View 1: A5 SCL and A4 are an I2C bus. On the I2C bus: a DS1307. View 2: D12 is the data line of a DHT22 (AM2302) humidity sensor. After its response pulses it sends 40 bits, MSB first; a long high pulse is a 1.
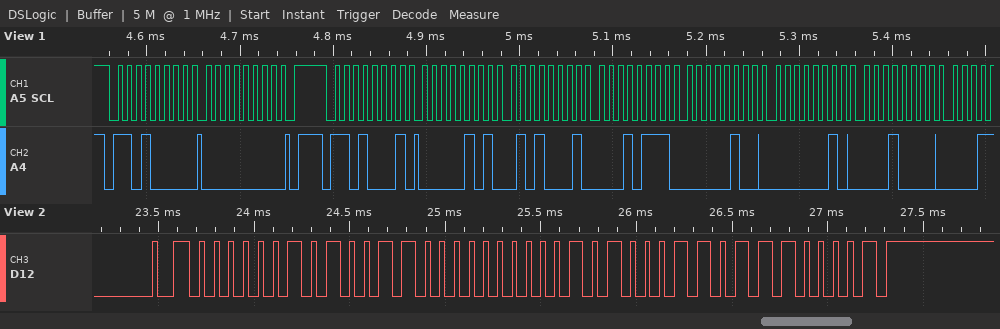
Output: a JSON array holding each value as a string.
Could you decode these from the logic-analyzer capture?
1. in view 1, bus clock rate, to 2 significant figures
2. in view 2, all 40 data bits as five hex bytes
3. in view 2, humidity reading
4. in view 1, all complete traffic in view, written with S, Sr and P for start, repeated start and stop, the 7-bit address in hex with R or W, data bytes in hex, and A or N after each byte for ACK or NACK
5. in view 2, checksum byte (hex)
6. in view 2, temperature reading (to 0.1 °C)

["100 kHz", "02 98 01 46 E1", "66.4 %", "S 68W A 00 A P S 68R A 05 A 51 A 17 A 04 A 02 A 10 A", "0xE1", "32.6 °C"]
